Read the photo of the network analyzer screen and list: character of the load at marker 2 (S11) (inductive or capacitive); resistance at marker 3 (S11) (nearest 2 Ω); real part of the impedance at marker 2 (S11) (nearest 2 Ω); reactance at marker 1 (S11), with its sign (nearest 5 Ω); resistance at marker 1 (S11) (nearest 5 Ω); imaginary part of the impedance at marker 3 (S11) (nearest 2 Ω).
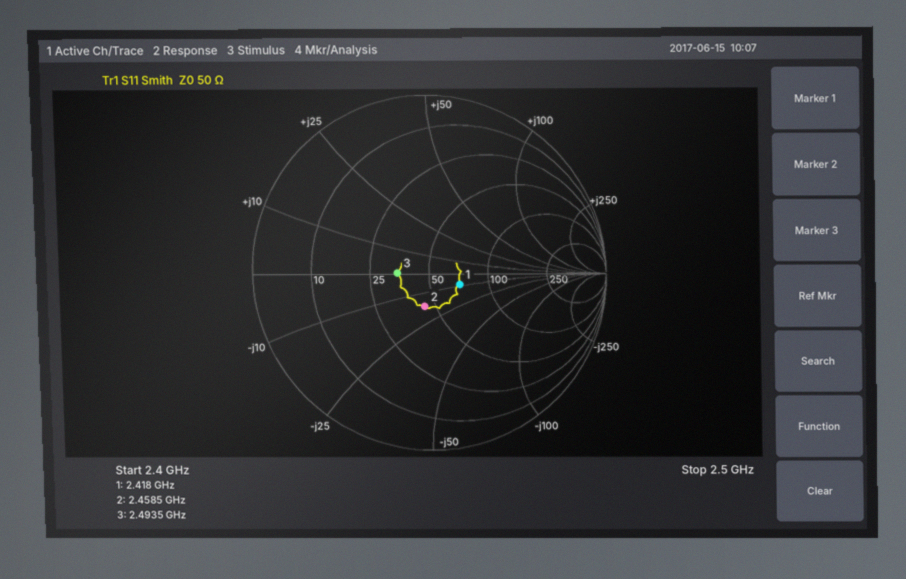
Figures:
capacitive
34 Ω
44 Ω
-10 Ω
70 Ω
0 Ω
